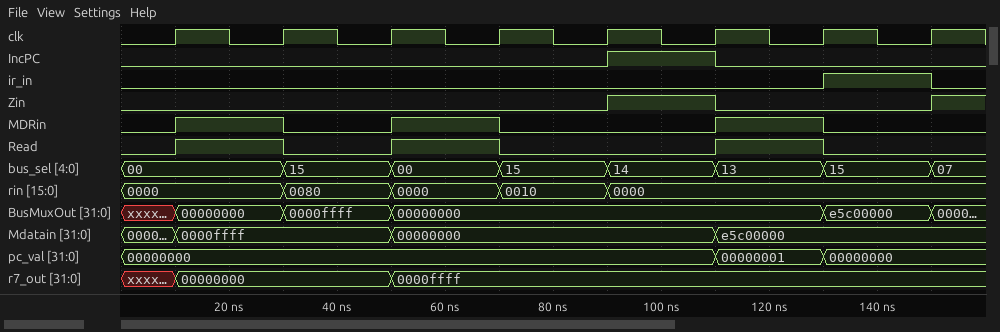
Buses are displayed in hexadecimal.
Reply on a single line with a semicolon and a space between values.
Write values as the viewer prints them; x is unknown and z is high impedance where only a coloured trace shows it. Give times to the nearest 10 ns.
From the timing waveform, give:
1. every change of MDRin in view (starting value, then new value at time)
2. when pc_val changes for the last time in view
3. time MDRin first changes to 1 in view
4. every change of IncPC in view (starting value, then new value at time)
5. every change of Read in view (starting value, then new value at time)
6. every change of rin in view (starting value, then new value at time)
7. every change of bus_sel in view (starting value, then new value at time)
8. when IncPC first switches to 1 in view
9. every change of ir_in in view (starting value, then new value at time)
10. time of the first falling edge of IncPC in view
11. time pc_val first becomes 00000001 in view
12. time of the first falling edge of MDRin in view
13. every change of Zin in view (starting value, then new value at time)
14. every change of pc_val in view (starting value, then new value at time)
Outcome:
0, 1 at 10 ns, 0 at 30 ns, 1 at 50 ns, 0 at 70 ns, 1 at 110 ns, 0 at 130 ns; 130 ns; 10 ns; 0, 1 at 90 ns, 0 at 110 ns; 0, 1 at 10 ns, 0 at 30 ns, 1 at 50 ns, 0 at 70 ns, 1 at 110 ns, 0 at 130 ns; 0000, 0080 at 30 ns, 0000 at 50 ns, 0010 at 70 ns, 0000 at 90 ns; 00, 15 at 30 ns, 00 at 50 ns, 15 at 70 ns, 14 at 90 ns, 13 at 110 ns, 15 at 130 ns, 07 at 150 ns; 90 ns; 0, 1 at 130 ns, 0 at 150 ns; 110 ns; 110 ns; 30 ns; 0, 1 at 90 ns, 0 at 110 ns, 1 at 150 ns; 00000000, 00000001 at 110 ns, 00000000 at 130 ns
